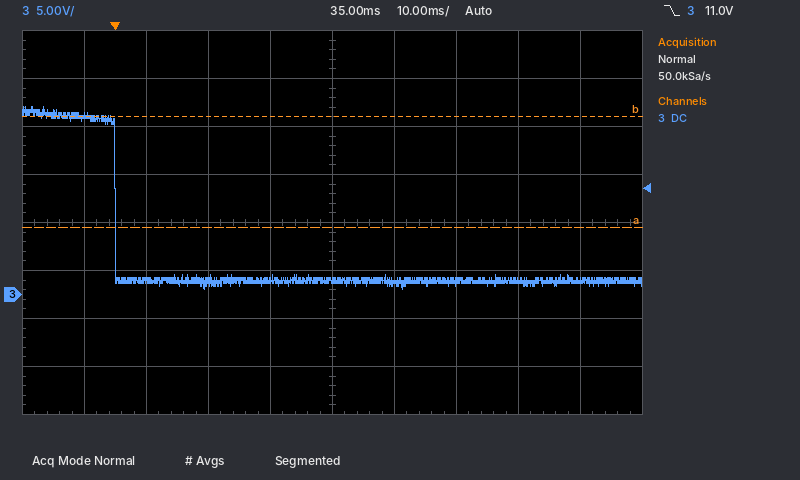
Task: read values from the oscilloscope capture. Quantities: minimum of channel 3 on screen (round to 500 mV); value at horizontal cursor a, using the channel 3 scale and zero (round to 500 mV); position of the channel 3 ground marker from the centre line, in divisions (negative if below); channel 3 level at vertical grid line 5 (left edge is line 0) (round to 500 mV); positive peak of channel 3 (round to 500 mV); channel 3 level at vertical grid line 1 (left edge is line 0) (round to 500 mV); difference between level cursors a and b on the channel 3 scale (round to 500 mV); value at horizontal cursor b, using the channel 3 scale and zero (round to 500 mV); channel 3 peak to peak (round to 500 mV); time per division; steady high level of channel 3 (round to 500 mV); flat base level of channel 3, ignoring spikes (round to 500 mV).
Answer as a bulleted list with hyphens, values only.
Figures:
- 500 mV
- 7.0 V
- -1.5 div
- 1.5 V
- 19.5 V
- 18.5 V
- 11.5 V
- 18.5 V
- 19.0 V
- 10 ms
- 18.5 V
- 1.5 V
